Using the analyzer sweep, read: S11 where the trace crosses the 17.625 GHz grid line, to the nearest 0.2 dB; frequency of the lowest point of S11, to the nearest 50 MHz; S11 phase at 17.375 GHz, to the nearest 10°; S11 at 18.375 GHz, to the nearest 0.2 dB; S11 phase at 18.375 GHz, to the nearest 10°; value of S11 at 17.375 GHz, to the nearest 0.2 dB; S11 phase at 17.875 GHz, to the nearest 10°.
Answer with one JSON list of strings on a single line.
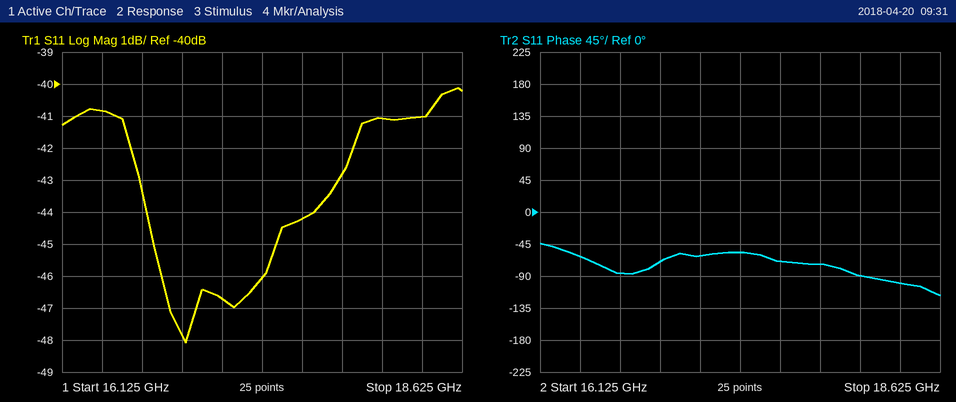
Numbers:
["-44.2 dB", "16.90 GHz", "-60°", "-41.0 dB", "-100°", "-46.0 dB", "-70°"]
